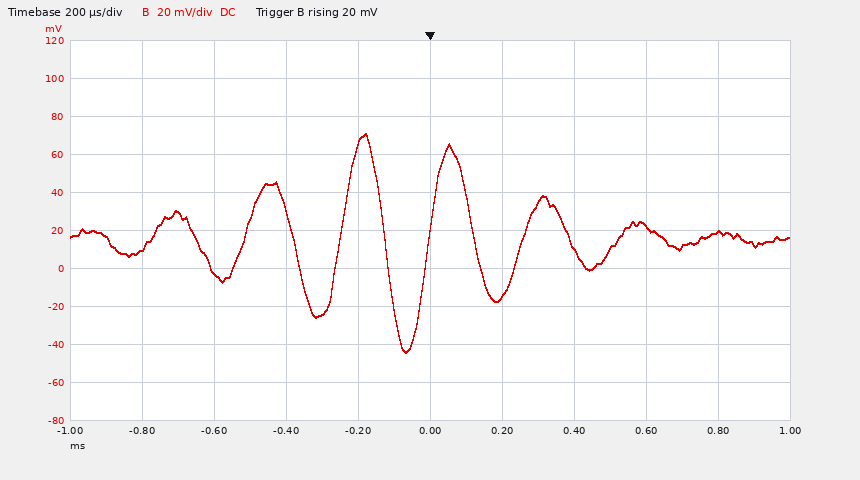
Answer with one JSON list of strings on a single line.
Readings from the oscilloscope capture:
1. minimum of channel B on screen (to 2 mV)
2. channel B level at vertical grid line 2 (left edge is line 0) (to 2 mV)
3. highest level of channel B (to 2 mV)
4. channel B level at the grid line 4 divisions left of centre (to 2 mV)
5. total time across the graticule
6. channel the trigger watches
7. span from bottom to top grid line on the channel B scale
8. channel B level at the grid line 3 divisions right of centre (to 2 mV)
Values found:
["-44 mV", "-2 mV", "72 mV", "10 mV", "2 ms", "channel B", "200 mV", "22 mV"]
